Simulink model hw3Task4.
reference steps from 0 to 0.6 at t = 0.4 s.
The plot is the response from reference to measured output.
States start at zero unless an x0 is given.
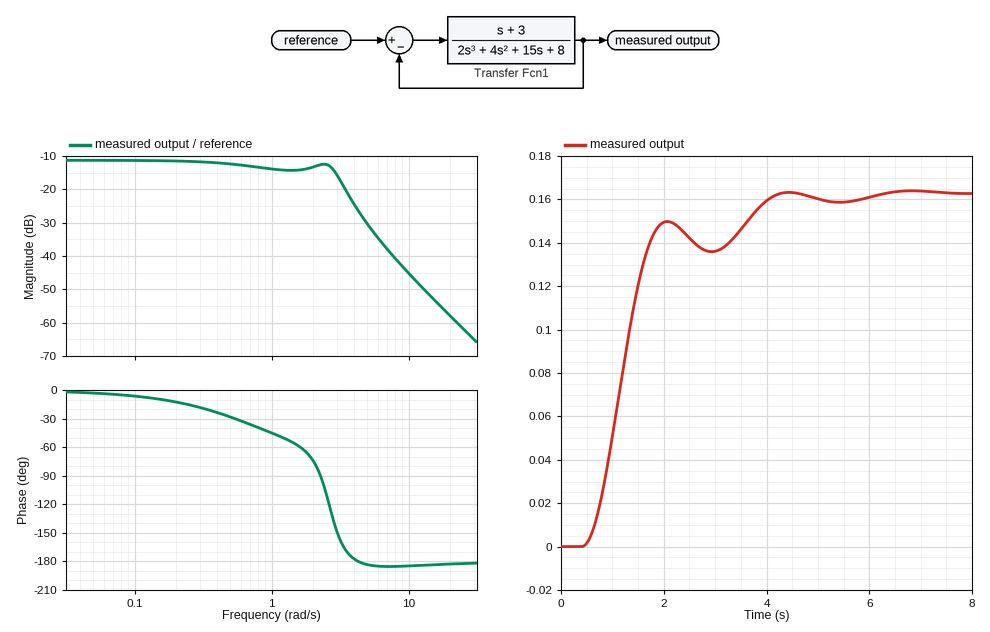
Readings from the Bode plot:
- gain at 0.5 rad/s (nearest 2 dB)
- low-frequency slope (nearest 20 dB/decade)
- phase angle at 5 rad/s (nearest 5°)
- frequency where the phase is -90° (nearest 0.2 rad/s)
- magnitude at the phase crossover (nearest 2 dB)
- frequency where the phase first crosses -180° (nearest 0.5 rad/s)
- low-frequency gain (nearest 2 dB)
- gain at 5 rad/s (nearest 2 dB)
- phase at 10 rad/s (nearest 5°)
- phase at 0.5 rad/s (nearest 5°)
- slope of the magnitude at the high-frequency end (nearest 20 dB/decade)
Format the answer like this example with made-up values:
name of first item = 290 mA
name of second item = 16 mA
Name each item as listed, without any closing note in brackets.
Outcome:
gain at 0.5 rad/s = -12 dB
low-frequency slope = 0 dB/decade
phase angle at 5 rad/s = -185°
frequency where the phase is -90° = 2.2 rad/s
magnitude at the phase crossover = -26 dB
frequency where the phase first crosses -180° = 4.5 rad/s
low-frequency gain = -12 dB
gain at 5 rad/s = -30 dB
phase at 10 rad/s = -185°
phase at 0.5 rad/s = -30°
slope of the magnitude at the high-frequency end = -40 dB/decade
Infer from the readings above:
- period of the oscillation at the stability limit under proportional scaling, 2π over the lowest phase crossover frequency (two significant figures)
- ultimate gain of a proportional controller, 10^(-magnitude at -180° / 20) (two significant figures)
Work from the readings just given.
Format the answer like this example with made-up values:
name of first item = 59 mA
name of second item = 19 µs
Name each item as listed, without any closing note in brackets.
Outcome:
period of the oscillation at the stability limit under proportional scaling, 2π over the lowest phase crossover frequency = 1.4 s
ultimate gain of a proportional controller, 10^(-magnitude at -180° / 20) = 20
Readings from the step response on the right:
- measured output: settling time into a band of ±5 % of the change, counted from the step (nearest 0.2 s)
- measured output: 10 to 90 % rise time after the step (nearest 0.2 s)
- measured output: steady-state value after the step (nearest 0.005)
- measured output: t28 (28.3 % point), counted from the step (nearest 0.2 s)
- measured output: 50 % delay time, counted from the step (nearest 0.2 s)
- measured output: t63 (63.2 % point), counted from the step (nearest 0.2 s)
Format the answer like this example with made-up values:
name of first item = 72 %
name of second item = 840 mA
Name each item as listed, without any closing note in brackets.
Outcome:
measured output: settling time into a band of ±5 % of the change, counted from the step = 3.4 s
measured output: 10 to 90 % rise time after the step = 1.2 s
measured output: steady-state value after the step = 0.165
measured output: t28 (28.3 % point), counted from the step = 0.6 s
measured output: 50 % delay time, counted from the step = 0.8 s
measured output: t63 (63.2 % point), counted from the step = 1.0 s
